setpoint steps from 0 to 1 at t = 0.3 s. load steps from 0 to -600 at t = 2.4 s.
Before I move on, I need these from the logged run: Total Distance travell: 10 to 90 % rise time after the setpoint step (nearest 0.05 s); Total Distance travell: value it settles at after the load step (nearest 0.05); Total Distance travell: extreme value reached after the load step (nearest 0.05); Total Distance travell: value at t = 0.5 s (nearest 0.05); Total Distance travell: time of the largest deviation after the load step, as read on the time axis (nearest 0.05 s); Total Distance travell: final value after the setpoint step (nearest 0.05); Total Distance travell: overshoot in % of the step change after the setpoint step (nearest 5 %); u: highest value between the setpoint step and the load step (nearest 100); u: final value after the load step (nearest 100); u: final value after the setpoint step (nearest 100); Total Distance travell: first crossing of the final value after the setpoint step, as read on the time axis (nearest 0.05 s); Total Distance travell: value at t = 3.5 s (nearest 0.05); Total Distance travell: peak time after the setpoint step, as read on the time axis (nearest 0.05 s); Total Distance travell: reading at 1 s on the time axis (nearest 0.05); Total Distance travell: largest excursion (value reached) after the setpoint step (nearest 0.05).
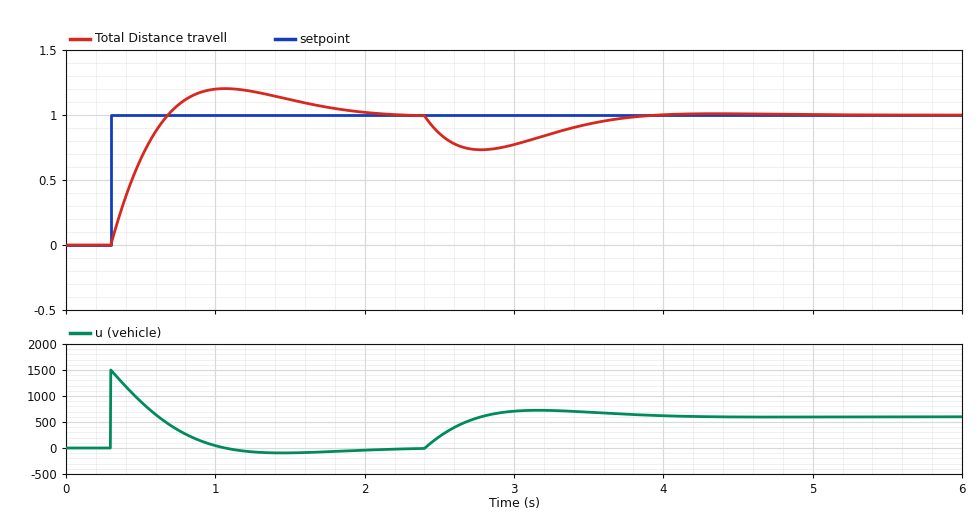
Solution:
0.30 s
1.00
0.75
0.65
2.80 s
1.00
20 %
1500
600
0
0.70 s
0.95
1.05 s
1.20
1.20
